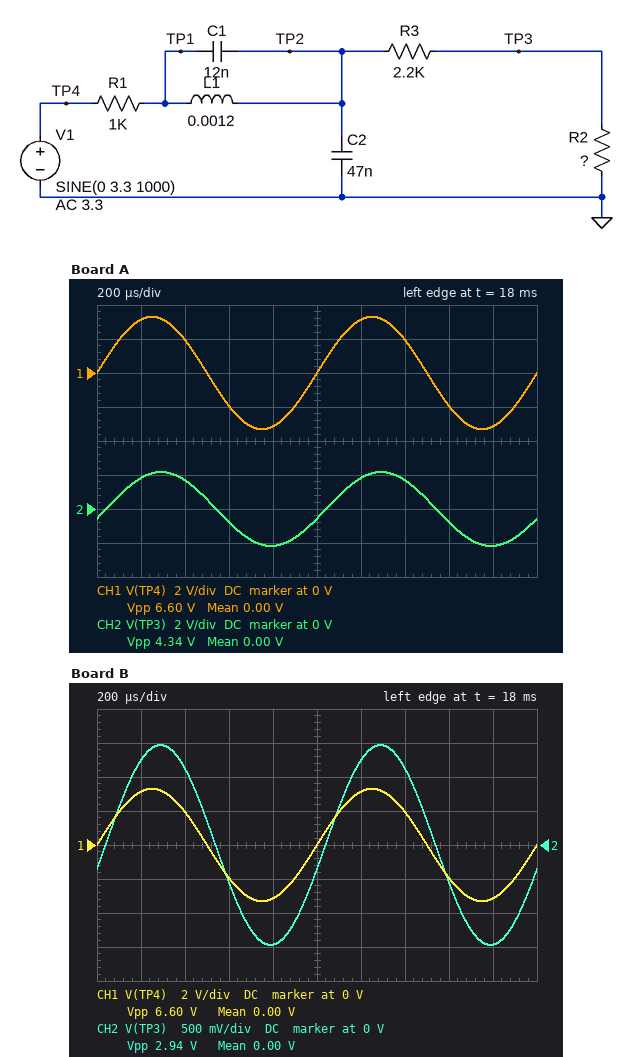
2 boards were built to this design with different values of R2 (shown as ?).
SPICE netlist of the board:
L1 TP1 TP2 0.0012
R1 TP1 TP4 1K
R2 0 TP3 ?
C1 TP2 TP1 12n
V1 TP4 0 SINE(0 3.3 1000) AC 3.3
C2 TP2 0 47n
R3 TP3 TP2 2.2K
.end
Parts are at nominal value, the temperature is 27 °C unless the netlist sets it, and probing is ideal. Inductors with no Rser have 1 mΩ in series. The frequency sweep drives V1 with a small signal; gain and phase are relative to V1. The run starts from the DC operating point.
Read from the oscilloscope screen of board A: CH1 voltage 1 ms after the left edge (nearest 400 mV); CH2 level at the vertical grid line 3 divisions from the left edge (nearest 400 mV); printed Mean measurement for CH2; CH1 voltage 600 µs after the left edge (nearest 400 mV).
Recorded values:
0 V
-800 mV
0.00 V
-2.0 V
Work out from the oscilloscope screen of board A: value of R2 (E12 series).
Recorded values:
6.8 kΩ
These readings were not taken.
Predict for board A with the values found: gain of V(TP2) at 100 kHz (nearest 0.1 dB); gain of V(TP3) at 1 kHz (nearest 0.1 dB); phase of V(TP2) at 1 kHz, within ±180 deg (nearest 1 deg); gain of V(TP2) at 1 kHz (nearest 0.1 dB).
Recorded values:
-29.6 dB
-3.6 dB
-15 deg
-1.2 dB
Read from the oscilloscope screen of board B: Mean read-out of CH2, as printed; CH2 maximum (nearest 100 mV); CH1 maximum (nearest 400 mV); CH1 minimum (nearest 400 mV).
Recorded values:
0.00 V
1.5 V
3.2 V
-3.2 V
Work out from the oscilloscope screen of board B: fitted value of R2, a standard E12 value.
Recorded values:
2.7 kΩ
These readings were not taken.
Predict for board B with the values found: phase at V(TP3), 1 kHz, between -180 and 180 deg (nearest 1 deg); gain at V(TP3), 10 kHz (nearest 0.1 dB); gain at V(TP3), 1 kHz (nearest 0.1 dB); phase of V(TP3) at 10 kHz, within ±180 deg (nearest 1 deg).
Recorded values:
-14 deg
-15.1 dB
-7.0 dB
-72 deg
